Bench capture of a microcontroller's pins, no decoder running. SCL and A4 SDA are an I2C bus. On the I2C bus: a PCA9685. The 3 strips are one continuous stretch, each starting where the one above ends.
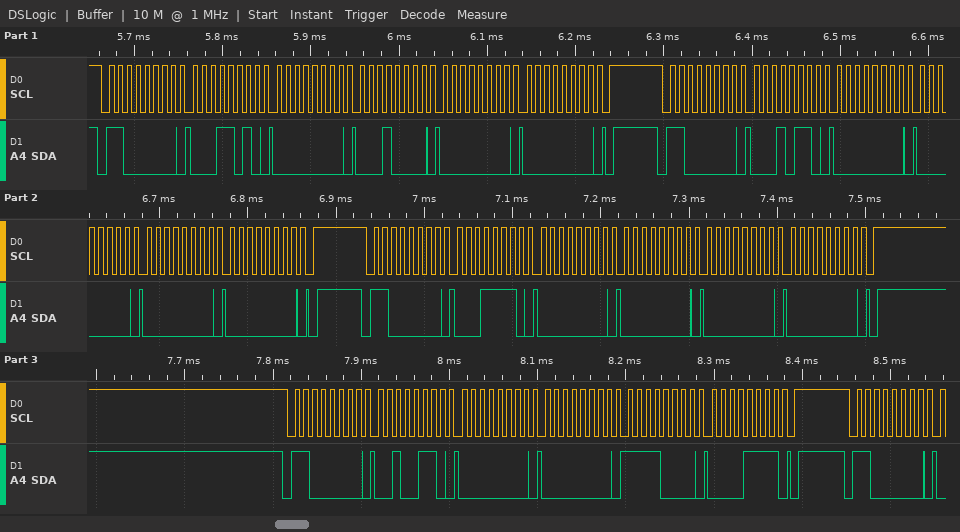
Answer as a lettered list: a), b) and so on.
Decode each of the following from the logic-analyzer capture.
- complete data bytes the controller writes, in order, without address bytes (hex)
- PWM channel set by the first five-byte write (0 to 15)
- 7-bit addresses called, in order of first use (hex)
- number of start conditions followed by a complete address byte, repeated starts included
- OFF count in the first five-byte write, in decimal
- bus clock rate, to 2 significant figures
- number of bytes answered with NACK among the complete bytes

a) 1A 00 10 00 00 16 00 00 00 00 1E 00 00 00 00 26 00 00 F0 0F
b) 5
c) 0x60
d) 5
e) 0
f) 100 kHz
g) 0
